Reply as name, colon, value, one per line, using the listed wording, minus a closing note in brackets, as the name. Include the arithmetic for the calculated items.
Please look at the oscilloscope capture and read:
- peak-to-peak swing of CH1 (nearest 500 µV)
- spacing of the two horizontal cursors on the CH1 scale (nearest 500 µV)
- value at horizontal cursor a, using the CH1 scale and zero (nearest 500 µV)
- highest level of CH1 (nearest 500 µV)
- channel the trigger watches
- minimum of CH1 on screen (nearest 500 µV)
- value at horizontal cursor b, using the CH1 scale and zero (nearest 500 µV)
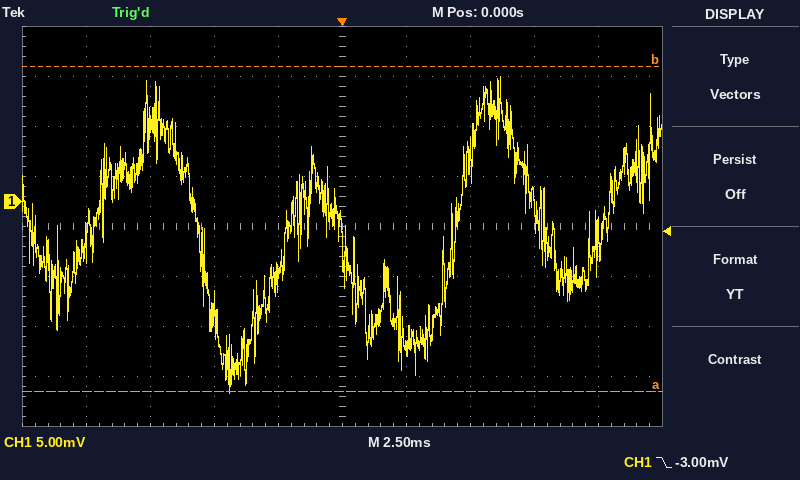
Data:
peak-to-peak swing of CH1: 12.5 mV − (-19.0 mV) = 31.5 mV
spacing of the two horizontal cursors on the CH1 scale: 32.5 mV
value at horizontal cursor a, using the CH1 scale and zero: -19.0 mV
highest level of CH1: 12.5 mV
channel the trigger watches: CH1
minimum of CH1 on screen: -19.0 mV
value at horizontal cursor b, using the CH1 scale and zero: 13.5 mV
